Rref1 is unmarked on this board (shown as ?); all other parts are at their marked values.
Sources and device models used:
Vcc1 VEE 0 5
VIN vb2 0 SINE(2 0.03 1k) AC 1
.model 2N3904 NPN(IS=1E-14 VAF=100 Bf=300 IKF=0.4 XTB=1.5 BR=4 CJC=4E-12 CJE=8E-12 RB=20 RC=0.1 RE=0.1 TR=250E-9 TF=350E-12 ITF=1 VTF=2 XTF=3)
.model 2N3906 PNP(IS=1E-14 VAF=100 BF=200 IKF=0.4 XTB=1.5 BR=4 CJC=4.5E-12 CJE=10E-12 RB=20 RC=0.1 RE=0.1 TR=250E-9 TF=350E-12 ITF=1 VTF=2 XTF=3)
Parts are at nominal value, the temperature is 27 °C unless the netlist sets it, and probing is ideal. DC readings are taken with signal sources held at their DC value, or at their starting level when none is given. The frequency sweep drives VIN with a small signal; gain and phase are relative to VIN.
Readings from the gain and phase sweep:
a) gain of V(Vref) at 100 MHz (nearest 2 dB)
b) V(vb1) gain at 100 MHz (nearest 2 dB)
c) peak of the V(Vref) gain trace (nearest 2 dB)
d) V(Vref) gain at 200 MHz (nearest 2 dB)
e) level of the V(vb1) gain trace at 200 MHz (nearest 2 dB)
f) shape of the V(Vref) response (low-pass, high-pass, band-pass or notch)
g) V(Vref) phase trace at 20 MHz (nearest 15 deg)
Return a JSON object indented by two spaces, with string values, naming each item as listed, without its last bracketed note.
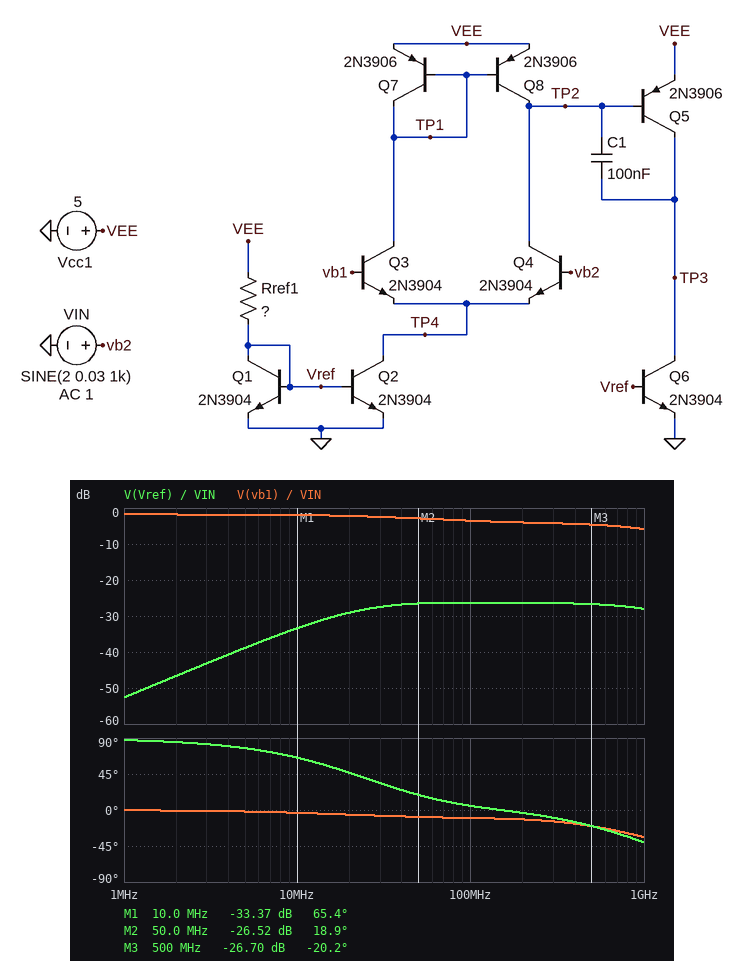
{
  "gain of V(Vref) at 100 MHz": "-26 dB",
  "V(vb1) gain at 100 MHz": "-4 dB",
  "peak of the V(Vref) gain trace": "-26 dB",
  "V(Vref) gain at 200 MHz": "-26 dB",
  "level of the V(vb1) gain trace at 200 MHz": "-4 dB",
  "shape of the V(Vref) response": "high-pass",
  "V(Vref) phase trace at 20 MHz": "45 deg"
}
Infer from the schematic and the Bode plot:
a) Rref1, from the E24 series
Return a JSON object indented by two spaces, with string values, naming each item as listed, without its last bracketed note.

{
  "Rref1, from the E24 series": "20 kΩ"
}
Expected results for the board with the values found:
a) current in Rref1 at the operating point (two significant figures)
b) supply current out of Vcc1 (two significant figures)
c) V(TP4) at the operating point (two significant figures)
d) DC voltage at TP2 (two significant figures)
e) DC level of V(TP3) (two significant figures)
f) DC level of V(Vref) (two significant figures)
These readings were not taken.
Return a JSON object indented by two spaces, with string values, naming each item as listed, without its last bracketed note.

{
  "current in Rref1 at the operating point": "220 µA",
  "supply current out of Vcc1": "660 µA",
  "V(TP4) at the operating point": "1.4 V",
  "DC voltage at TP2": "4.3 V",
  "DC level of V(TP3)": "5.0 V",
  "DC level of V(Vref)": "620 mV"
}
